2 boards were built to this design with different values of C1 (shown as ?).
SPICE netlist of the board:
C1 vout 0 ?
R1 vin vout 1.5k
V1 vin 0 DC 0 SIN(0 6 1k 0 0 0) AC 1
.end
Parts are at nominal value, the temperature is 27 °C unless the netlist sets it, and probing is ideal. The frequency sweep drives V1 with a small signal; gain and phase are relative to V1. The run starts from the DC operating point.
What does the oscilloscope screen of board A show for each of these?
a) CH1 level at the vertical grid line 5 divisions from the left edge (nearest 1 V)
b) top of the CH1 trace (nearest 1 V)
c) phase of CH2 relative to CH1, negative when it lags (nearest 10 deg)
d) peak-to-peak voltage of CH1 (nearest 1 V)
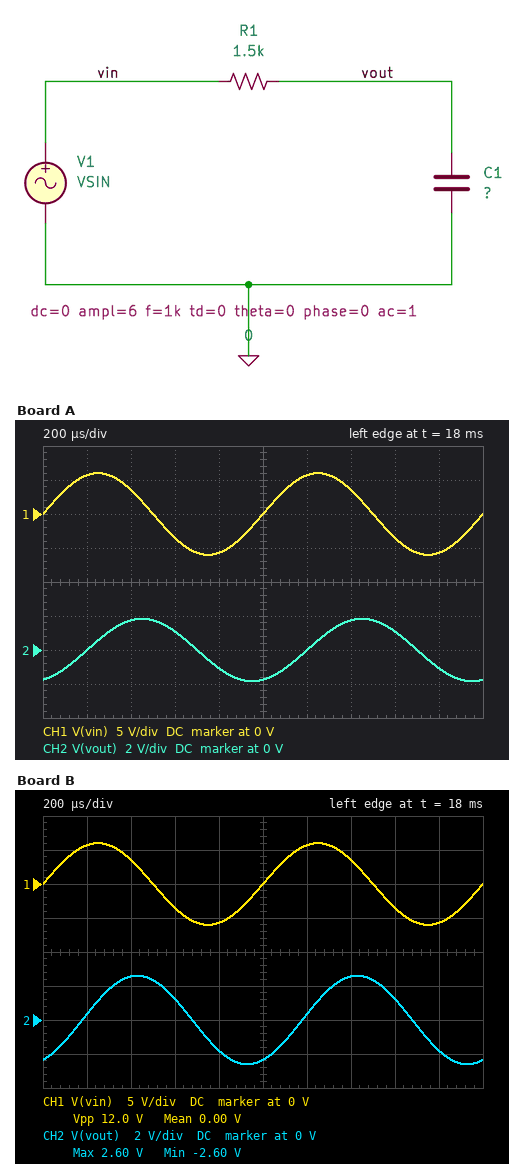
0 V
6 V
-70 deg
12 V
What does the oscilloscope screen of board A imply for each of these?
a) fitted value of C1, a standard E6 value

330 nF
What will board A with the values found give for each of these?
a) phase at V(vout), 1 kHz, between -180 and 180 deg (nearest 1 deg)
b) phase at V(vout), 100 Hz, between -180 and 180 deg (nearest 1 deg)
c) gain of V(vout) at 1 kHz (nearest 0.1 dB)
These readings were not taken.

-72 deg
-17 deg
-10.3 dB
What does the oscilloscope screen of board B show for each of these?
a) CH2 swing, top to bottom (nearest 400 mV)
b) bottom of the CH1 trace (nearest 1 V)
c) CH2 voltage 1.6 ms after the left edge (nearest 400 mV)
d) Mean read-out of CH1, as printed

5.2 V
-6 V
1.2 V
0.00 V
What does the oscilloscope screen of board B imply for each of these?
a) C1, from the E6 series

220 nF
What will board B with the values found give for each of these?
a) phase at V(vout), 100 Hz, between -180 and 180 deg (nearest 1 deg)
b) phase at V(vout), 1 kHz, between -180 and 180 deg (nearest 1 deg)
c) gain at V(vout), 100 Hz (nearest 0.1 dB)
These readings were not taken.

-12 deg
-64 deg
-0.2 dB
